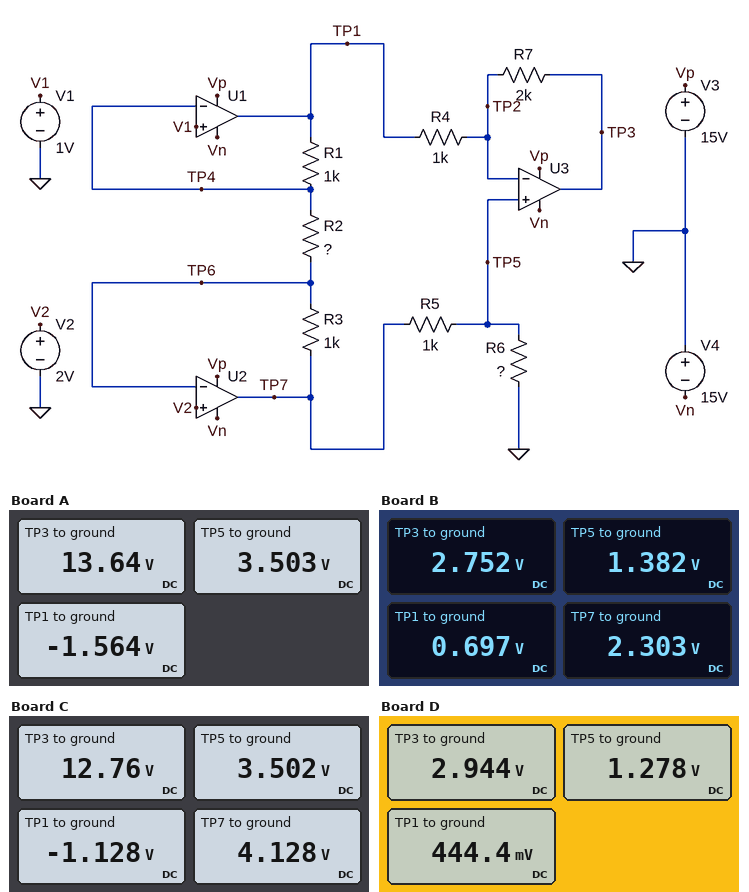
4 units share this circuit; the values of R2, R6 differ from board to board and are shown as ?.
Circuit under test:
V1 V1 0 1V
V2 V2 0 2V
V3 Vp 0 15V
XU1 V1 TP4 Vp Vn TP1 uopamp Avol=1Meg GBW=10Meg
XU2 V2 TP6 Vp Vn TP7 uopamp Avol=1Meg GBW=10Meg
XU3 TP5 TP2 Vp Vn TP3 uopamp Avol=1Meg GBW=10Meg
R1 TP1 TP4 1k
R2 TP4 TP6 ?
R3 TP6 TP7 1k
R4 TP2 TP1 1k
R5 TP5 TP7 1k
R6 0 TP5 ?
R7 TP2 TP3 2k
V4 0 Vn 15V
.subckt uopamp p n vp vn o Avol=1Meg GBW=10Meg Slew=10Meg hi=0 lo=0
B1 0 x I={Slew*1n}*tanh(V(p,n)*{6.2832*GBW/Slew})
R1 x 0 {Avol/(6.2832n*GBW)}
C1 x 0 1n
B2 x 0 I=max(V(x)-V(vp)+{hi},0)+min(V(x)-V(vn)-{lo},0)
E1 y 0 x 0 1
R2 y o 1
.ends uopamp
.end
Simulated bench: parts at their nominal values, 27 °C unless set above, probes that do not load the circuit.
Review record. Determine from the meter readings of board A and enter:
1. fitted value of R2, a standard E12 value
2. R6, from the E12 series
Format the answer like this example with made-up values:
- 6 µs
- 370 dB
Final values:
- 390 Ω
- 3.3 kΩ
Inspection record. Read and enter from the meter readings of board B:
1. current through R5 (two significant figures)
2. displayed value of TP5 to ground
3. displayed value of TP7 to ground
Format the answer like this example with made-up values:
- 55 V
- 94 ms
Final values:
- 920 µA
- 1.382 V
- 2.303 V
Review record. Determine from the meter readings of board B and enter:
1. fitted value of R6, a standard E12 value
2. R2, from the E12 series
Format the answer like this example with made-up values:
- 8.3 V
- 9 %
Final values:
- 1.5 kΩ
- 3.3 kΩ
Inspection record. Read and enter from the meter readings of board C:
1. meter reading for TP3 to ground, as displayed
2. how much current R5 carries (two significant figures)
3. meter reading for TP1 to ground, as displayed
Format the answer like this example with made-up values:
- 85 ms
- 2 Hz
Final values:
- 12.76 V
- 630 µA
- -1.128 V
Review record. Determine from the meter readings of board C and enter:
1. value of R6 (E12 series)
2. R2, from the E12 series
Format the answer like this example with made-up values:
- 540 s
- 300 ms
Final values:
- 5.6 kΩ
- 470 Ω
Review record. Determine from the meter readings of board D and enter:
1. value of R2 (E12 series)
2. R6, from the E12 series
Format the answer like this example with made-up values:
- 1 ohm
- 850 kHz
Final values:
- 1.8 kΩ
- 1 kΩ
